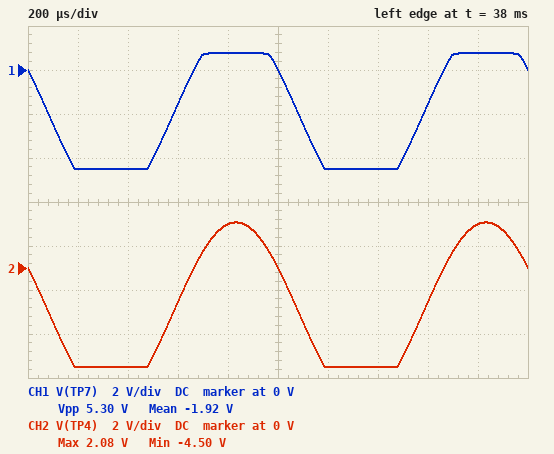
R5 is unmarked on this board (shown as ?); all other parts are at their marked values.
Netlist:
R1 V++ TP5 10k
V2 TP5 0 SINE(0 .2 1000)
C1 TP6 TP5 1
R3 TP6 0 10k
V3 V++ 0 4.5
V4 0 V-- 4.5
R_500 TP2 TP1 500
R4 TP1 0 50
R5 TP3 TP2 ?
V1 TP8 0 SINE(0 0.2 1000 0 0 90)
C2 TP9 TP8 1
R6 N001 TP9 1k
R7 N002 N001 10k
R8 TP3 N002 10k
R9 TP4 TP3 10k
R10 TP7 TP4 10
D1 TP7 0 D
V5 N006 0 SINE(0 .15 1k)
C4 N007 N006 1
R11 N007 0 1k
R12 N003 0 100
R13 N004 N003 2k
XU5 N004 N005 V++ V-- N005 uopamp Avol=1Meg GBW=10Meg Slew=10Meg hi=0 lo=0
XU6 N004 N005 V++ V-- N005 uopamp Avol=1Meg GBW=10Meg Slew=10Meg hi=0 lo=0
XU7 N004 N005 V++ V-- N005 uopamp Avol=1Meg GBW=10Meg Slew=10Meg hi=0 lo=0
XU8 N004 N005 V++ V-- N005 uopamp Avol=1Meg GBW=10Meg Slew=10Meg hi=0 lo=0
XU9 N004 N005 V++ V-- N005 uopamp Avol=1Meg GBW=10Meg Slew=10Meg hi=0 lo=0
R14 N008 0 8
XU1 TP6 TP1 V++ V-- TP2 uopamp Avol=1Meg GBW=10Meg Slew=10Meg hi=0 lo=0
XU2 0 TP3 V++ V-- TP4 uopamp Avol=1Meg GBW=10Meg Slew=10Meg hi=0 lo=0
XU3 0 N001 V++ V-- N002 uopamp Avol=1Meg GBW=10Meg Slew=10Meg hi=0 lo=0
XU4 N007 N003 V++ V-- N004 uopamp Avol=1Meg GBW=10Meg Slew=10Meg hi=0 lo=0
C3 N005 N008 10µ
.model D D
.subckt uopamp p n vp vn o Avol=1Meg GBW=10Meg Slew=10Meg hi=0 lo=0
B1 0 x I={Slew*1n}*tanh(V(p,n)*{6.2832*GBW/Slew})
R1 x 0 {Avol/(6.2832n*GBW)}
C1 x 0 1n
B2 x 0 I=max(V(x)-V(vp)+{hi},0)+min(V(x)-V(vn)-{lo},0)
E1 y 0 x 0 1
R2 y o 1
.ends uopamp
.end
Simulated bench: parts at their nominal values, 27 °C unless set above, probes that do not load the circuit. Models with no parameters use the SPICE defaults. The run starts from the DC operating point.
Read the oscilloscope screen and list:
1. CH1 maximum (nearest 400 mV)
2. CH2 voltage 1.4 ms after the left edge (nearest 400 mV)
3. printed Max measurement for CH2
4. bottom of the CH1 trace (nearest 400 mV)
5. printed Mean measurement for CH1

800 mV
-4.4 V
2.08 V
-4.4 V
-1.92 V
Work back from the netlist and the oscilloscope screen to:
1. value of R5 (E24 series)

6.2 kΩ
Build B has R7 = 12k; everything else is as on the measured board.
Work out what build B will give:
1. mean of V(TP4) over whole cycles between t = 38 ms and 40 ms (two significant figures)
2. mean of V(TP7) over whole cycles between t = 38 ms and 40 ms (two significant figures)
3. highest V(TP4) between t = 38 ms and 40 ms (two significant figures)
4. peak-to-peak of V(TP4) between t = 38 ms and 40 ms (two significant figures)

-1.9 V
-2.1 V
1.9 V
6.4 V
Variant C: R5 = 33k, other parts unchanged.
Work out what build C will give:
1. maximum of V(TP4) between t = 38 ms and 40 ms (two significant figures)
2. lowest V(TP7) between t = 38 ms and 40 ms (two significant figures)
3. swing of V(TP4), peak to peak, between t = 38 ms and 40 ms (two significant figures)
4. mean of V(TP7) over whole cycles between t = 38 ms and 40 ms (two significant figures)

110 mV
-4.1 V
4.2 V
-2.0 V
